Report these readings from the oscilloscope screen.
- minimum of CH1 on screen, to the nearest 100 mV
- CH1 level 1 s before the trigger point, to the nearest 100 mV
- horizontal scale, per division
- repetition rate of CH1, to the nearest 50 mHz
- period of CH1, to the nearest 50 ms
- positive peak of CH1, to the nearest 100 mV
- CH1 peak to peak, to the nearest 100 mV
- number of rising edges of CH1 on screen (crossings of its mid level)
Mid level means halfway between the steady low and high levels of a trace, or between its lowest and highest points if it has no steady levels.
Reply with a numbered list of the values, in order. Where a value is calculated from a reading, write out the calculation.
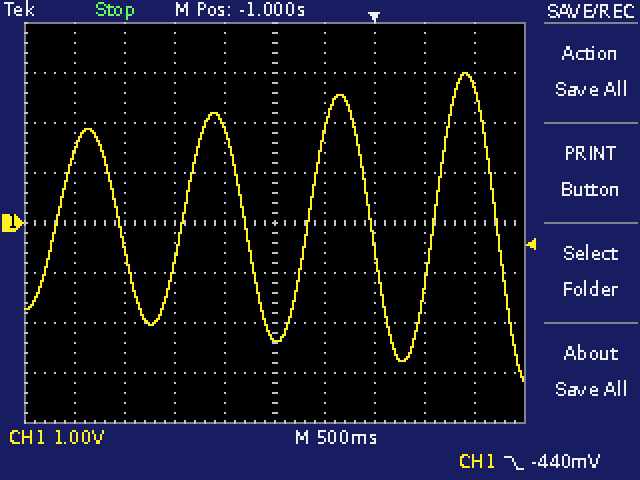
1. -3.2 V
2. -2.3 V
3. 500 ms
4. 1 / 1.25 s ≈ 800 mHz
5. 1.25 s
6. 3.0 V
7. 3.0 V − (-3.2 V) = 6.2 V
8. 4
